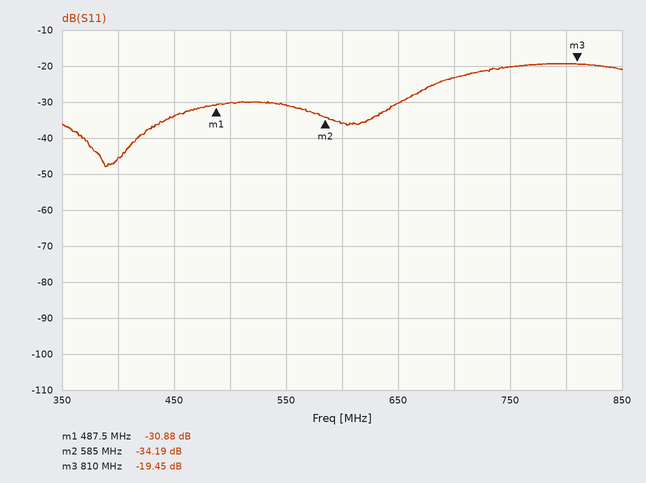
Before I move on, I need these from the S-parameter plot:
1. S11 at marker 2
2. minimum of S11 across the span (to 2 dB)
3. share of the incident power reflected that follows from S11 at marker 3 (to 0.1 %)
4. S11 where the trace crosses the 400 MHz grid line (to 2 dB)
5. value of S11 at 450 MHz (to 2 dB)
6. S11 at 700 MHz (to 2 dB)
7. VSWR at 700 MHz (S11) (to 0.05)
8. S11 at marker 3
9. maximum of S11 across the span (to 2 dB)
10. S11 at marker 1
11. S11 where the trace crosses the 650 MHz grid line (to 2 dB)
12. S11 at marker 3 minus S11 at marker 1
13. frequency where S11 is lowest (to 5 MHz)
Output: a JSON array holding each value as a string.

["-34.19 dB", "-48 dB", "1.1 %", "-46 dB", "-34 dB", "-24 dB", "1.15", "-19.45 dB", "-20 dB", "-30.88 dB", "-30 dB", "11.43 dB", "390 MHz"]
